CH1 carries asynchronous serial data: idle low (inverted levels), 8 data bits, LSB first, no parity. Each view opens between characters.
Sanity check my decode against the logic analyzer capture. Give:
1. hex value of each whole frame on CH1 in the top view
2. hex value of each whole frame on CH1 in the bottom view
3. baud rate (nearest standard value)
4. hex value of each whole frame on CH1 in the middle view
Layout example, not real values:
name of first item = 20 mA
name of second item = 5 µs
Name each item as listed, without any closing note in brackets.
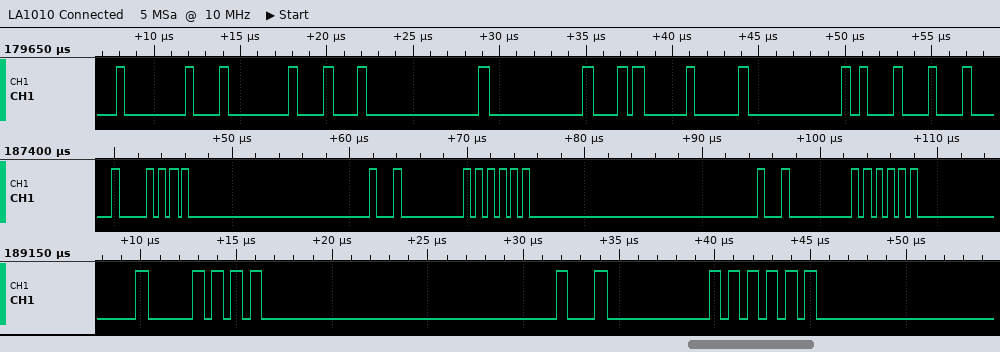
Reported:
hex value of each whole frame on CH1 in the top view = 7F, 7F, F7, FF, D7, DF, DD
hex value of each whole frame on CH1 in the bottom view = 5F, FD, F7, 55, FF
baud rate = 2000000 baud
hex value of each whole frame on CH1 in the middle view = 5F, FD, F7, 55, FF, F7, 55, FF
